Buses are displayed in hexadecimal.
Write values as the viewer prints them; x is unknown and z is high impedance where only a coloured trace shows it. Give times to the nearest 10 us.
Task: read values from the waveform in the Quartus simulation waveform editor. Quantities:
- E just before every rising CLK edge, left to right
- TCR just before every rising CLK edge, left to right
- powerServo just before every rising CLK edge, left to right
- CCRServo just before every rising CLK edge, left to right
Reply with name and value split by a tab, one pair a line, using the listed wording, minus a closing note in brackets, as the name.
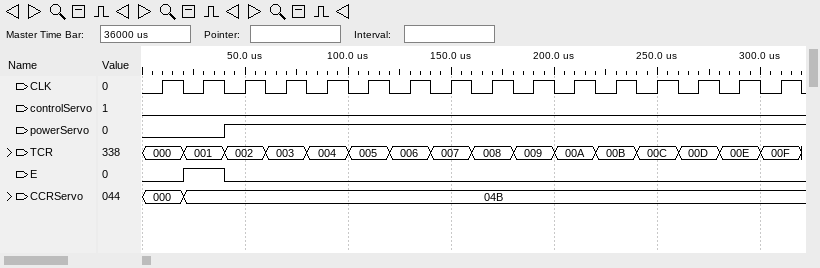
E just before every rising CLK edge, left to right	0 1 0 0 0 0 0 0 0 0 0 0 0 0 0 0
TCR just before every rising CLK edge, left to right	000, 001, 002, 003, 004, 005, 006, 007, 008, 009, 00A, 00B, 00C, 00D, 00E, 00F
powerServo just before every rising CLK edge, left to right	0 0 1 1 1 1 1 1 1 1 1 1 1 1 1 1
CCRServo just before every rising CLK edge, left to right	000, 04B, 04B, 04B, 04B, 04B, 04B, 04B, 04B, 04B, 04B, 04B, 04B, 04B, 04B, 04B
